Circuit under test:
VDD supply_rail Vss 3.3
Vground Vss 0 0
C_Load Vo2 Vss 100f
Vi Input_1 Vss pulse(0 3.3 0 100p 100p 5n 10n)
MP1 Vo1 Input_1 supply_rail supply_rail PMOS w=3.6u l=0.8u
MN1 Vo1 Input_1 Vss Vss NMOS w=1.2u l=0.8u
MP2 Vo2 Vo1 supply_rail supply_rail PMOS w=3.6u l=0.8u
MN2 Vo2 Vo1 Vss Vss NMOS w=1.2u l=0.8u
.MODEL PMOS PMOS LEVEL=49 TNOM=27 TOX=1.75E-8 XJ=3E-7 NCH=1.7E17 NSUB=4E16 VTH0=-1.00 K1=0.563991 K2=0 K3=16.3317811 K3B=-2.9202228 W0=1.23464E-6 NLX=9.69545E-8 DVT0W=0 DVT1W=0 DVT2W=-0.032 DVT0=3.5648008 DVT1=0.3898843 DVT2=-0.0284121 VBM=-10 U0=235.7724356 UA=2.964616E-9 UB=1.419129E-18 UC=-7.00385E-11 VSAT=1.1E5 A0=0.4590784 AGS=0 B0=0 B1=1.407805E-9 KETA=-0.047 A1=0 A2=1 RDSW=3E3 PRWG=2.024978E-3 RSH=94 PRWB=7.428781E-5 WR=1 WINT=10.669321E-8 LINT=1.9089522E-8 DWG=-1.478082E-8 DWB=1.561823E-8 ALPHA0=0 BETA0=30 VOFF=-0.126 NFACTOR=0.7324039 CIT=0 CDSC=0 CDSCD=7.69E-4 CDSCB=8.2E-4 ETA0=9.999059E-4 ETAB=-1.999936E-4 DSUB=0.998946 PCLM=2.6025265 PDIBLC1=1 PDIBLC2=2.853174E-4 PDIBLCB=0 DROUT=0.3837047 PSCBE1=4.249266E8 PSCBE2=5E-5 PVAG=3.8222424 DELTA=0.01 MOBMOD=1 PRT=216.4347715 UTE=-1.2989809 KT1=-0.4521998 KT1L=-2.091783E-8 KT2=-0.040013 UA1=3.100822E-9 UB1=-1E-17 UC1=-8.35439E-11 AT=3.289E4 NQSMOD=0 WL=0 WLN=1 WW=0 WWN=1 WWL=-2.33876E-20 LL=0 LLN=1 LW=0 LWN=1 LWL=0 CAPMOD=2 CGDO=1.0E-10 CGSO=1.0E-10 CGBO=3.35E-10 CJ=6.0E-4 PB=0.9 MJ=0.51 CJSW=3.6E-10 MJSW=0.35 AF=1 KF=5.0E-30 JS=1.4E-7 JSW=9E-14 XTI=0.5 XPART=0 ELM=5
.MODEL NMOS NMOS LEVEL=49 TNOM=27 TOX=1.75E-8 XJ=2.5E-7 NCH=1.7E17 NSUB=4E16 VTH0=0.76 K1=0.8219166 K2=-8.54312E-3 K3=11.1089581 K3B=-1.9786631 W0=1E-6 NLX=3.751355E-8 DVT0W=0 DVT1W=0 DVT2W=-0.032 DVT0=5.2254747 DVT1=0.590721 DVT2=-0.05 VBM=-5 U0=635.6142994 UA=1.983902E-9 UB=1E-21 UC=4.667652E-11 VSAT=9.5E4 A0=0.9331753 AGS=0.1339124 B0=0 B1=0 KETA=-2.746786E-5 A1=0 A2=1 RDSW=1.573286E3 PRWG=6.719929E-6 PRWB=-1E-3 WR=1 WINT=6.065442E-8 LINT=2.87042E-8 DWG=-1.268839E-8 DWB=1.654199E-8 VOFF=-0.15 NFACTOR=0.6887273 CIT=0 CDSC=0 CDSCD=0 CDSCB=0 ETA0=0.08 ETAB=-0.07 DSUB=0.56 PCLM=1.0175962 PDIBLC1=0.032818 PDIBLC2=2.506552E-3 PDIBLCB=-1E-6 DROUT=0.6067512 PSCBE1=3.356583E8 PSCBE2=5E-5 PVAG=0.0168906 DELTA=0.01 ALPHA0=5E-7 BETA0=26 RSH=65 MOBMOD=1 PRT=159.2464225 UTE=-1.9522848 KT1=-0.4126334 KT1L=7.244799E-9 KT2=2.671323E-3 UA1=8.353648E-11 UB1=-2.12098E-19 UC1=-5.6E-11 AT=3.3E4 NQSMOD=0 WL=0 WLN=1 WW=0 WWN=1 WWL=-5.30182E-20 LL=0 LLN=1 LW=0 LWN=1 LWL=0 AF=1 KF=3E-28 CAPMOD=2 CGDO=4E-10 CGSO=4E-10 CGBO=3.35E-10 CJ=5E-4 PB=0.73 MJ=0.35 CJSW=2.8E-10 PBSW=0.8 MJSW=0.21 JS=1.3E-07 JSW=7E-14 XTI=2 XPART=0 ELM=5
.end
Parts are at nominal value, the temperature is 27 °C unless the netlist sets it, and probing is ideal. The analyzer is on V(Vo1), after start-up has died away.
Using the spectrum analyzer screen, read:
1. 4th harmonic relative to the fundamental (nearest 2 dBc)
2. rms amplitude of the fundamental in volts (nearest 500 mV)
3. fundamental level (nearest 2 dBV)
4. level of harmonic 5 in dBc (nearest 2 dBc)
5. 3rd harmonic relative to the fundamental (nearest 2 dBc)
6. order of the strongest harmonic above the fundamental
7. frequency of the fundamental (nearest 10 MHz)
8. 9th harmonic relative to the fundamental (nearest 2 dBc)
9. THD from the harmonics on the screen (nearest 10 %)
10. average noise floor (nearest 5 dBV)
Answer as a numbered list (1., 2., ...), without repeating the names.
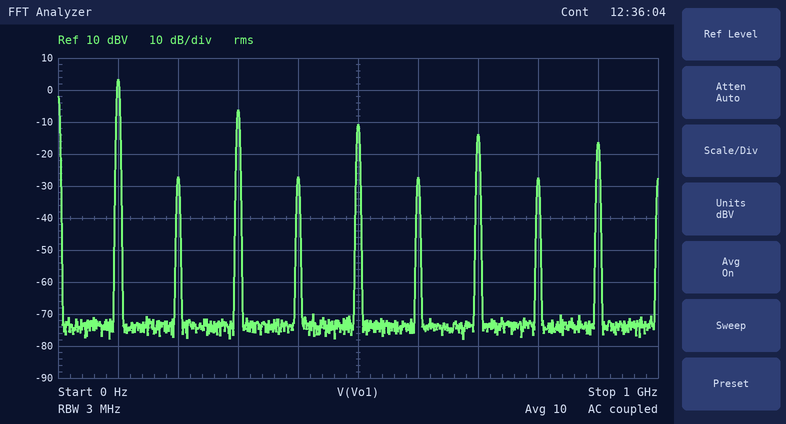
1. -30 dBc
2. 1.5 V
3. 4 dBV
4. -14 dBc
5. -10 dBc
6. 3
7. 100 MHz
8. -20 dBc
9. 40 %
10. -75 dBV
